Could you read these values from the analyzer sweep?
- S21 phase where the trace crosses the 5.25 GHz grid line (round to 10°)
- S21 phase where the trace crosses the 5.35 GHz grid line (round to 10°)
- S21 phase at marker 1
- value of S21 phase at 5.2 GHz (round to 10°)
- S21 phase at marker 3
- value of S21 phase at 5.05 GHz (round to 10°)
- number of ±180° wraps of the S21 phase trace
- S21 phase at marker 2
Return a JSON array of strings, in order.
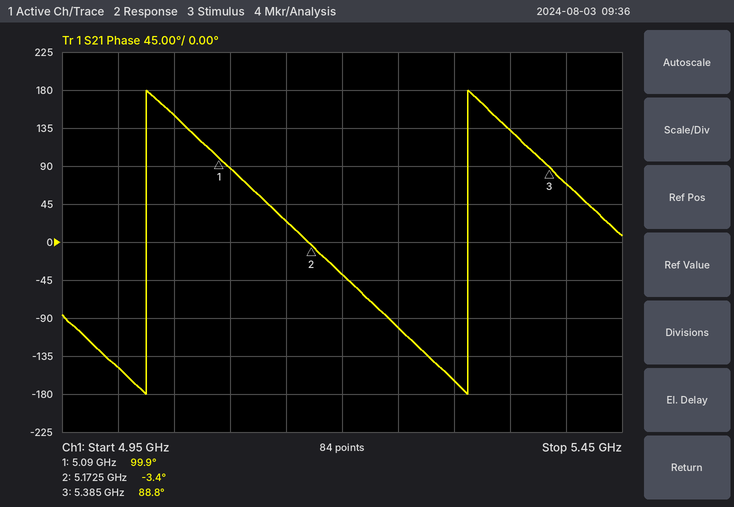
["-100°", "130°", "99.9°", "-40°", "88.8°", "150°", "2", "-3.4°"]
